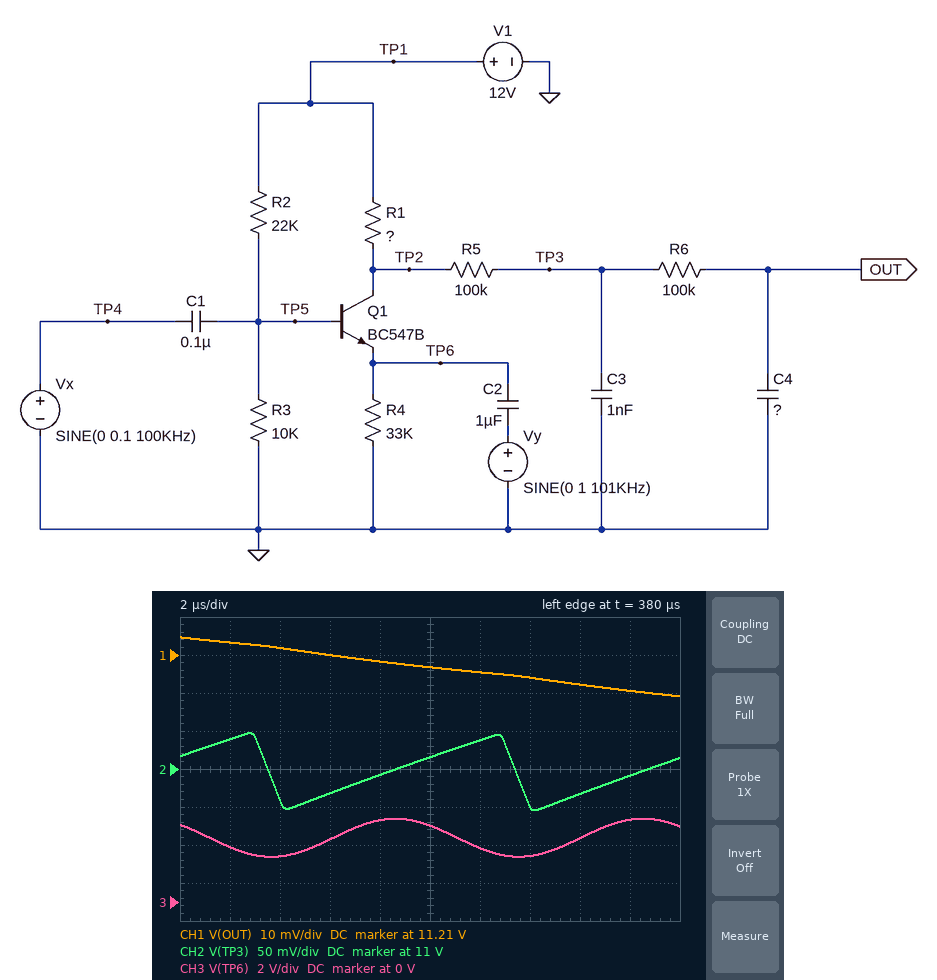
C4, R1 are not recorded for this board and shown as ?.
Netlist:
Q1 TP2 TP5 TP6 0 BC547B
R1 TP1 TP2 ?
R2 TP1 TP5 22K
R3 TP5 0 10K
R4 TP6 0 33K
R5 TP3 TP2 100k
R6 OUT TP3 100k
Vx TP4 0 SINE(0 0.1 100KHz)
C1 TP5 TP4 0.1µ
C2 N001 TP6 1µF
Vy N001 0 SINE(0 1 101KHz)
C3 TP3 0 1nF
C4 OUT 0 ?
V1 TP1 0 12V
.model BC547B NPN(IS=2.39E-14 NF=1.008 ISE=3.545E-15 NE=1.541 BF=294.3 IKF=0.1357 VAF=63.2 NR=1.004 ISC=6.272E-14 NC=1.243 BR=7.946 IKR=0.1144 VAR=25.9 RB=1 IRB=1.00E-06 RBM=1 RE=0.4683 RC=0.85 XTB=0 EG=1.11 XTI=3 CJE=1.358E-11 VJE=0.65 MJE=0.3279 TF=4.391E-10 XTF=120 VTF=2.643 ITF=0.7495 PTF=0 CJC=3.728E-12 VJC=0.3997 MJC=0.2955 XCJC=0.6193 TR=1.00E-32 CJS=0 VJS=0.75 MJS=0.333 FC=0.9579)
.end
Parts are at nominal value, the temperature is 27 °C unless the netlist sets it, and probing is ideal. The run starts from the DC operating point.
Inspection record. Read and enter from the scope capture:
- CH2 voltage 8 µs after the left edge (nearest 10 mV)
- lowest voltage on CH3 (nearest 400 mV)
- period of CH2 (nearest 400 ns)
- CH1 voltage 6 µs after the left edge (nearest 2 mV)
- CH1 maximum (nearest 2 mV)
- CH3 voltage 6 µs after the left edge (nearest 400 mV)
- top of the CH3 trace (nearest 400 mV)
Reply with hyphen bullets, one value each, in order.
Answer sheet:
- 10.99 V
- 2.4 V
- 10.0 µs
- 11.210 V
- 11.214 V
- 3.2 V
- 4.4 V
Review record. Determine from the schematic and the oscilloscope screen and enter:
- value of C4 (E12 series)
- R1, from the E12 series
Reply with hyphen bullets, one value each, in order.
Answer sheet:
- 2.7 nF
- 3.9 kΩ
